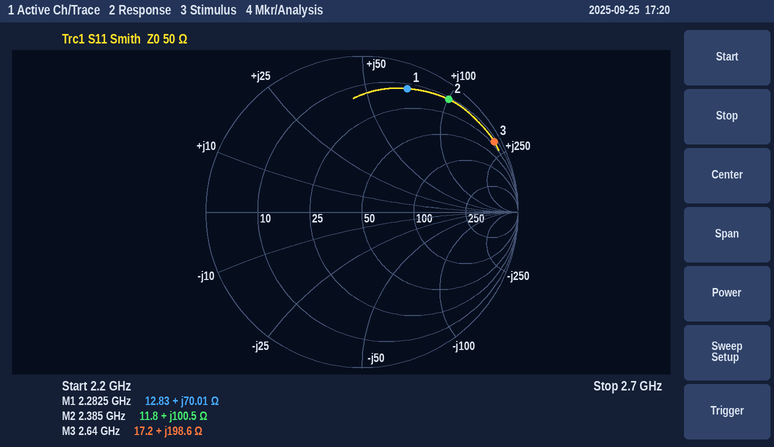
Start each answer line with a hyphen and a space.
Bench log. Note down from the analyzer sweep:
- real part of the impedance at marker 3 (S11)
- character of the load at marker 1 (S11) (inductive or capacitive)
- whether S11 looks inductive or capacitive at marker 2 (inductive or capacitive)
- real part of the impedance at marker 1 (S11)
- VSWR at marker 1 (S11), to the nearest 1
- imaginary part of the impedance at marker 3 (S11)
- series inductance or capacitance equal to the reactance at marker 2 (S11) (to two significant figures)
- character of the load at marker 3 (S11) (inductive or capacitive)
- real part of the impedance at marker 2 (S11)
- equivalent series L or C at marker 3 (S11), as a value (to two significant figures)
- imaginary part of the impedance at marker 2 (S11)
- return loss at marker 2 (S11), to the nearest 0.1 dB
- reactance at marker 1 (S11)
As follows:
- 17.2 Ω
- inductive
- inductive
- 12.83 Ω
- 12
- +198.6 Ω
- 6.7 nH
- inductive
- 11.8 Ω
- 12 nH
- +100.5 Ω
- 0.8 dB
- +70.01 Ω
